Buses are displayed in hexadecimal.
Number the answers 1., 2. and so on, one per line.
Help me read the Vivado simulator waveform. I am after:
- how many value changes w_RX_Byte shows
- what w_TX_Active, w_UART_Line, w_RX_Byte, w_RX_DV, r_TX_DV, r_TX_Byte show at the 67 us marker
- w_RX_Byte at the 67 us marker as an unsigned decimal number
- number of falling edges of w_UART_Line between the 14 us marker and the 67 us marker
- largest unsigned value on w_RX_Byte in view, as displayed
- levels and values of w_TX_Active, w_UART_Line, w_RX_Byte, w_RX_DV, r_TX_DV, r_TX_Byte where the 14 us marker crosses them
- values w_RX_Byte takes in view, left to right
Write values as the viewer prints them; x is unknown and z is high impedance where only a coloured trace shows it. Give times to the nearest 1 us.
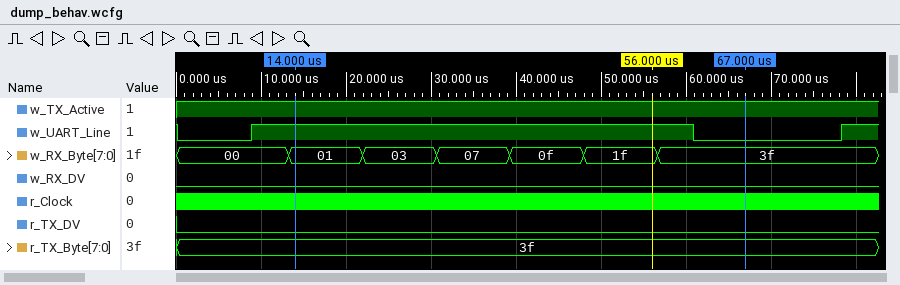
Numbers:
1. 6
2. w_TX_Active=1, w_UART_Line=0, w_RX_Byte=3f, w_RX_DV=0, r_TX_DV=0, r_TX_Byte=3f
3. 63
4. 1
5. 3f
6. w_TX_Active=1, w_UART_Line=1, w_RX_Byte=01, w_RX_DV=0, r_TX_DV=0, r_TX_Byte=3f
7. 00, 01, 03, 07, 0f, 1f, 3f
